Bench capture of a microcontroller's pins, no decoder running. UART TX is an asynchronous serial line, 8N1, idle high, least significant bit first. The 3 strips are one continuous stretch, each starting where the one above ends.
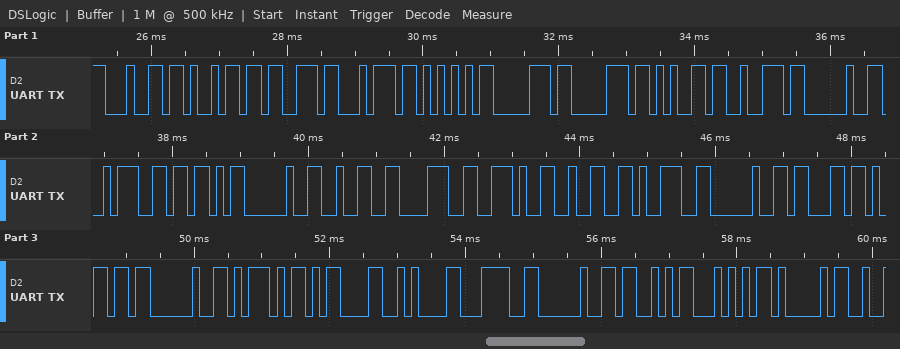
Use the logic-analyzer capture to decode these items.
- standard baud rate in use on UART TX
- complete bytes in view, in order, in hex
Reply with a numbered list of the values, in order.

1. 9600 baud
2. 64 69 73 74 55 70 70 65 72 20 3A 5B 20 32 38 2E 32 39 20 63 6D 20 5D 0D 0A 3C 20 53 54 41
